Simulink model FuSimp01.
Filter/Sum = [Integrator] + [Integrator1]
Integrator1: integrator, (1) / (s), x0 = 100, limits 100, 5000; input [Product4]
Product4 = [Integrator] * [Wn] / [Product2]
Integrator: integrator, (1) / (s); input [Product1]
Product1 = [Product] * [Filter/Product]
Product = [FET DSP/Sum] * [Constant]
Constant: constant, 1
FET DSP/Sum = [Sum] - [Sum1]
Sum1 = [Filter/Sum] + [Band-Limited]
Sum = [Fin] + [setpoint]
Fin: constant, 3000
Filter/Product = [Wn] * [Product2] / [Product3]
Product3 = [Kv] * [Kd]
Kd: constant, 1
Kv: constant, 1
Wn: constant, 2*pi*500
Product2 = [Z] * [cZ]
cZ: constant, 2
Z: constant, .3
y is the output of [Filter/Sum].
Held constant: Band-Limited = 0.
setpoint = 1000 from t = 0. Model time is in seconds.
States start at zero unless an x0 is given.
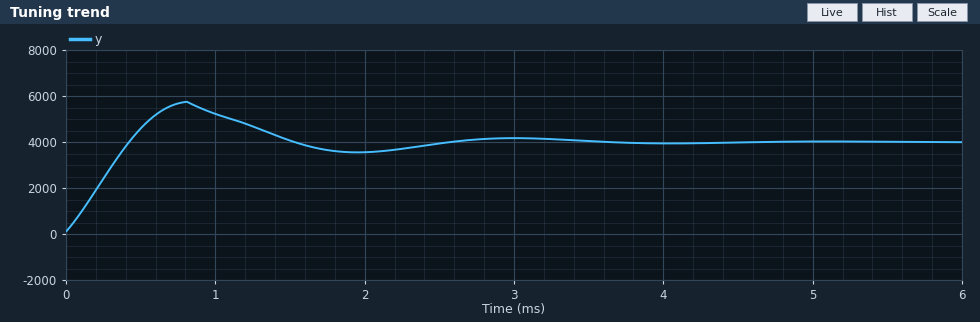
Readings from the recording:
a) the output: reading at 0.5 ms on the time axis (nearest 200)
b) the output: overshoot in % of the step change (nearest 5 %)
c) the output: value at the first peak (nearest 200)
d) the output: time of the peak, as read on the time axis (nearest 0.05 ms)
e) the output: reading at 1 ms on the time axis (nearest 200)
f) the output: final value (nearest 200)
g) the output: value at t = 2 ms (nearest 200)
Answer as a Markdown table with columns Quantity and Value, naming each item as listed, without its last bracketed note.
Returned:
| Quantity | Value |
|---|---|
| the output: reading at 0.5 ms on the time axis | 4600 |
| the output: overshoot in % of the step change | 45 % |
| the output: value at the first peak | 5800 |
| the output: time of the peak, as read on the time axis | 0.80 ms |
| the output: reading at 1 ms on the time axis | 5200 |
| the output: final value | 4000 |
| the output: value at t = 2 ms | 3600 |
